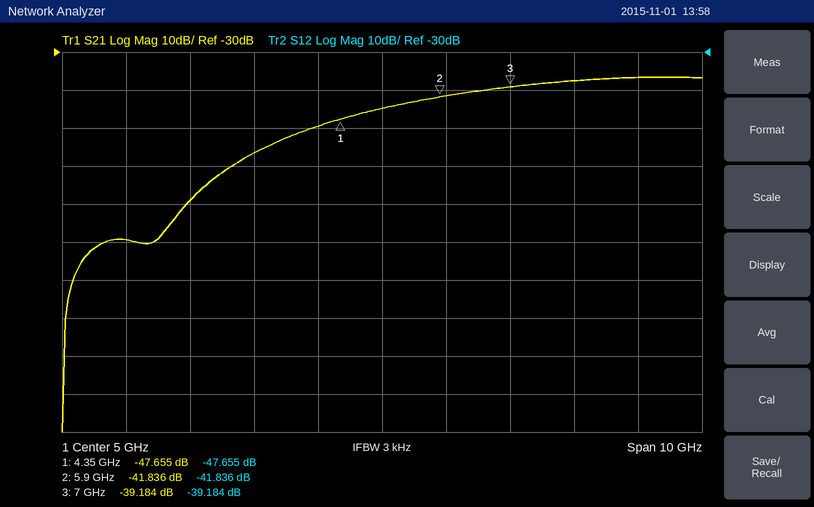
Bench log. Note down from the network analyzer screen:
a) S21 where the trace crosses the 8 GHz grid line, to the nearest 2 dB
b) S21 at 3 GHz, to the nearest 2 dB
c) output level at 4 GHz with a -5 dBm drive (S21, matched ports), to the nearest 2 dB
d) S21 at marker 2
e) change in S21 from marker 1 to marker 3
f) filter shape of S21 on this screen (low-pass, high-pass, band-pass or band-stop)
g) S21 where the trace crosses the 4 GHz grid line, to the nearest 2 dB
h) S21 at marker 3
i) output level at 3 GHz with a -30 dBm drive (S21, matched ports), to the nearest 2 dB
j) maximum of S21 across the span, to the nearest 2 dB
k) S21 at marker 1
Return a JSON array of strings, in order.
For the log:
["-38 dB", "-56 dB", "-54 dBm", "-41.836 dB", "8.471 dB", "high-pass", "-50 dB", "-39.184 dB", "-86 dBm", "-36 dB", "-47.655 dB"]
